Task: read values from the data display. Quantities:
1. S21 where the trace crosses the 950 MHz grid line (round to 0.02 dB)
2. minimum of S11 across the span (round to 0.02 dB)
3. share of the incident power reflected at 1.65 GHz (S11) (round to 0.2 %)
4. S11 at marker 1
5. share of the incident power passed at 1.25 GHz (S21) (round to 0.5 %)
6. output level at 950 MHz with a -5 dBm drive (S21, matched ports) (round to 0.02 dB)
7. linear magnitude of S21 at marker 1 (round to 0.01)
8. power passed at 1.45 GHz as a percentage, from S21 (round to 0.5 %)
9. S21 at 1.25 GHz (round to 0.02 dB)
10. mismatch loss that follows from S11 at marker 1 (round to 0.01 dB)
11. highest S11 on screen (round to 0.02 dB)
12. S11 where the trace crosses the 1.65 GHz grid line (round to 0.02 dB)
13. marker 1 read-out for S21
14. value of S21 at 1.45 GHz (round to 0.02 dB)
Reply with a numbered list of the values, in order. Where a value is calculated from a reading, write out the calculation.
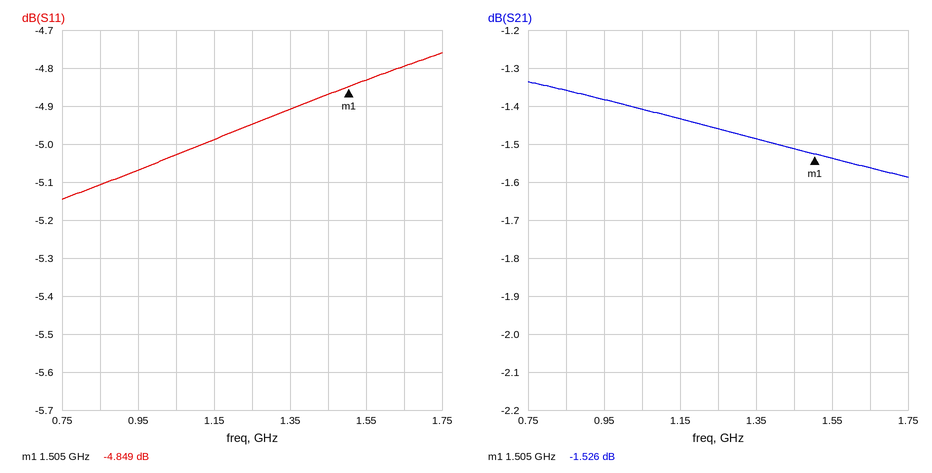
1. -1.38 dB
2. -5.14 dB
3. 10^(-4.8/10) ≈ 33.1 %, so 33.2 % to the nearest 0.2 %
4. -4.849 dB
5. 10^(-1.46/10) ≈ 71.4 %, so 71.5 % to the nearest 0.5 %
6. -5 dBm + (-1.38 dB) = -6.38 dBm
7. 10^(-1.526/20) ≈ 0.84
8. 10^(-1.52/10) ≈ 70.5 %
9. -1.46 dB
10. −10 log10(1 − 10^(-4.849/10)) ≈ 1.72 dB
11. -4.76 dB
12. -4.80 dB
13. -1.526 dB
14. -1.52 dB
